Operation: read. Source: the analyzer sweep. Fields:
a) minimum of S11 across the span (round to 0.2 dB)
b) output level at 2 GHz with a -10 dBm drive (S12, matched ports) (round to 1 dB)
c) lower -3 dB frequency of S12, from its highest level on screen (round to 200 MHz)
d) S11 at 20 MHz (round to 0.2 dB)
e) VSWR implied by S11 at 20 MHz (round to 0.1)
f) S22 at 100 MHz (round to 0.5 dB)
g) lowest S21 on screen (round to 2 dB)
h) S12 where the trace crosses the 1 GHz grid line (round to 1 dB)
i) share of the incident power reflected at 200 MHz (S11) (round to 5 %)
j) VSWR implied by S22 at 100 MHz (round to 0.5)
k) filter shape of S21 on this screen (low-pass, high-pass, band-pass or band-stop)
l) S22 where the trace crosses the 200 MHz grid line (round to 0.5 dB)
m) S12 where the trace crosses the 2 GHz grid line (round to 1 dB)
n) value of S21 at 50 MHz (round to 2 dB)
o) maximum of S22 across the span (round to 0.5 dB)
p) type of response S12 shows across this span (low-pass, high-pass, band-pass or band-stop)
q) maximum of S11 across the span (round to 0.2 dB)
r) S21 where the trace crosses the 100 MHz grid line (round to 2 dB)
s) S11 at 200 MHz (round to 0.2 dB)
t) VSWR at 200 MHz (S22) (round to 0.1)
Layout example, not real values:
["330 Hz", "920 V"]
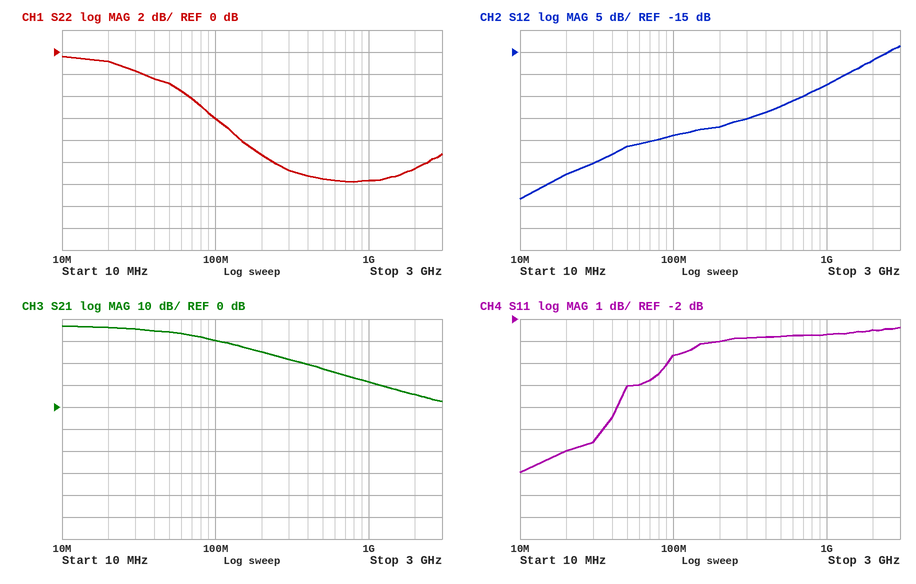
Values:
["-9.0 dB", "-27 dBm", "2.0 GHz", "-8.0 dB", "2.3", "-6.0 dB", "2 dB", "-22 dB", "50 %", "3.0", "low-pass", "-9.5 dB", "-17 dB", "34 dB", "-0.5 dB", "high-pass", "-2.4 dB", "30 dB", "-3.0 dB", "2.0"]
